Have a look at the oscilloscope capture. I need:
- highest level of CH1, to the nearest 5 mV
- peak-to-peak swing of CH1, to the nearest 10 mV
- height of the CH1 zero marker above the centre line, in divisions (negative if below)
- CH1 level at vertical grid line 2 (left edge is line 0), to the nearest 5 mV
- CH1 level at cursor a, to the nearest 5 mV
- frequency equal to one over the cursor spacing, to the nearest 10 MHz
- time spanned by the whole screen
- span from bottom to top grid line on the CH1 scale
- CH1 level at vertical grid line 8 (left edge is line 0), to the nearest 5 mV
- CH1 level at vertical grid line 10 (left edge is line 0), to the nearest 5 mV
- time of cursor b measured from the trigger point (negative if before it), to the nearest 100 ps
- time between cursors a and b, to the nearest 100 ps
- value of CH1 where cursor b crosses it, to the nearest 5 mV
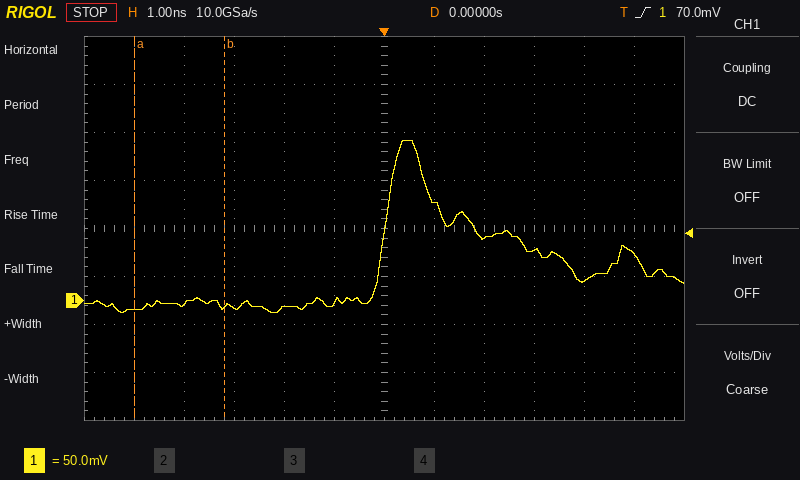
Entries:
165 mV
180 mV
-1.5 div
-5 mV
-10 mV
560 MHz
12 ns
400 mV
65 mV
20 mV
-3.2 ns
1.8 ns
-5 mV
